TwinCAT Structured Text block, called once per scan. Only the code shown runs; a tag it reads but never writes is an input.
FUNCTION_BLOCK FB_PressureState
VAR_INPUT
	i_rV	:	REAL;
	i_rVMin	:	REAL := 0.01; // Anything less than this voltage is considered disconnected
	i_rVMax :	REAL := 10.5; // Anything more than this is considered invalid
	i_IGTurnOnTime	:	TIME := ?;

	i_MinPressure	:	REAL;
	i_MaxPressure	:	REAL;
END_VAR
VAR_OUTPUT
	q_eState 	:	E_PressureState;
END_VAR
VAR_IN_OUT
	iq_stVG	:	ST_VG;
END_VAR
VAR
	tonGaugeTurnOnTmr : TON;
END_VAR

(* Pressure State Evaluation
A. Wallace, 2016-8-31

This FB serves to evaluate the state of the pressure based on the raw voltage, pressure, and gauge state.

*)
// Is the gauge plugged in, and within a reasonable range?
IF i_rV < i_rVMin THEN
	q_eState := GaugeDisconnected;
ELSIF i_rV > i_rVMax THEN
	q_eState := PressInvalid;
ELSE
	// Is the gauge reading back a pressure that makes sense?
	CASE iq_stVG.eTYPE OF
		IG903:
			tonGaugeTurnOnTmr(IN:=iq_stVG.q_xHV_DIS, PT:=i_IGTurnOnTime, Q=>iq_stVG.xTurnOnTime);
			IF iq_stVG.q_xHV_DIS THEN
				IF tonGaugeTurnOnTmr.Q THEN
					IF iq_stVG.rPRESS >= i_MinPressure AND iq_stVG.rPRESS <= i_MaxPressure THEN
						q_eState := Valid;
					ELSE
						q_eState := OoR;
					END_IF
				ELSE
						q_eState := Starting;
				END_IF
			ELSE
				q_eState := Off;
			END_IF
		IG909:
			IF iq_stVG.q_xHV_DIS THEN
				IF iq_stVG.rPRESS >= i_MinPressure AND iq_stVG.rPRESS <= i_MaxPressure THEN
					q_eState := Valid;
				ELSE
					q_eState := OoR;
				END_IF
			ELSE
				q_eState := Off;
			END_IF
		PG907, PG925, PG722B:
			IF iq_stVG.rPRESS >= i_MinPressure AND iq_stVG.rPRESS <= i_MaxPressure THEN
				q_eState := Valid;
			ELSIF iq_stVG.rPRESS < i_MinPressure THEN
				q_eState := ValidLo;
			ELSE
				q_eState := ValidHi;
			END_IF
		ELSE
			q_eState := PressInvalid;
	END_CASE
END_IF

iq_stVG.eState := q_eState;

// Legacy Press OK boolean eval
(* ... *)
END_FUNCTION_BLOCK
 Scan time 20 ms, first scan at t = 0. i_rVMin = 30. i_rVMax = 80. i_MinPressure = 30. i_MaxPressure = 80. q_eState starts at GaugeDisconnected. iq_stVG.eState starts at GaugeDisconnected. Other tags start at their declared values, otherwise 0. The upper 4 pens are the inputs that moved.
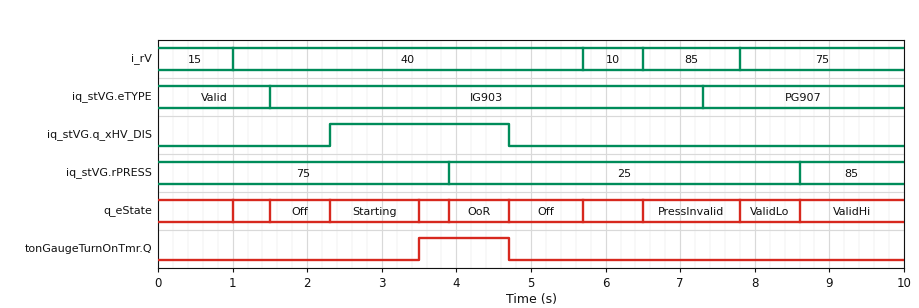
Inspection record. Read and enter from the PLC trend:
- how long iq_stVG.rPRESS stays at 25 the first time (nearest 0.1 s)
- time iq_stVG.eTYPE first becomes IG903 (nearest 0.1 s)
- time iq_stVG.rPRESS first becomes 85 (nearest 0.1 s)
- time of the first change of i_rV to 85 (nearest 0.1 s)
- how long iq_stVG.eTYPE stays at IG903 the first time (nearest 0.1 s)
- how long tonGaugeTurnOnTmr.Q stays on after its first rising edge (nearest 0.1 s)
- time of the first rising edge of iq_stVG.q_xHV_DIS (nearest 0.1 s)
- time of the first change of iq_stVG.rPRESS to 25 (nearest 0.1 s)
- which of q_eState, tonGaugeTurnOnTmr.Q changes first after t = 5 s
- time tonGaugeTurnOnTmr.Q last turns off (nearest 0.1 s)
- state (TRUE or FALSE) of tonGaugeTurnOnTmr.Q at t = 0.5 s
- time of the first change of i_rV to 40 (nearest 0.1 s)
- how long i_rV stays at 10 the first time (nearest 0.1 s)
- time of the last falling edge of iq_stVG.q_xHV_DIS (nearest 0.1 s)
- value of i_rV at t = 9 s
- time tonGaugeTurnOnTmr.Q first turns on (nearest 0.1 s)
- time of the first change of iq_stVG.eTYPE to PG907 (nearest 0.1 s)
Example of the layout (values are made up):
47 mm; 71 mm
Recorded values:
4.7 s; 1.5 s; 8.6 s; 6.5 s; 5.8 s; 1.2 s; 2.3 s; 3.9 s; q_eState; 4.7 s; FALSE; 1.0 s; 0.8 s; 4.7 s; 75; 3.5 s; 7.3 s
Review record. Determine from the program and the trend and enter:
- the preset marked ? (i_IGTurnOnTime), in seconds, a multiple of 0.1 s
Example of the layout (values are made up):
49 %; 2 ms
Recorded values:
1.2 s
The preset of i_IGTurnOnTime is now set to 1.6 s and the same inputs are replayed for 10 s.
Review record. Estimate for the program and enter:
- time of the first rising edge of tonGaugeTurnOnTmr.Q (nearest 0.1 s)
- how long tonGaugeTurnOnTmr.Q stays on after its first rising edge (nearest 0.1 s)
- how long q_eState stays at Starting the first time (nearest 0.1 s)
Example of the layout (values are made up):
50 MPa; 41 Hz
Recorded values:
3.9 s; 0.8 s; 1.6 s
